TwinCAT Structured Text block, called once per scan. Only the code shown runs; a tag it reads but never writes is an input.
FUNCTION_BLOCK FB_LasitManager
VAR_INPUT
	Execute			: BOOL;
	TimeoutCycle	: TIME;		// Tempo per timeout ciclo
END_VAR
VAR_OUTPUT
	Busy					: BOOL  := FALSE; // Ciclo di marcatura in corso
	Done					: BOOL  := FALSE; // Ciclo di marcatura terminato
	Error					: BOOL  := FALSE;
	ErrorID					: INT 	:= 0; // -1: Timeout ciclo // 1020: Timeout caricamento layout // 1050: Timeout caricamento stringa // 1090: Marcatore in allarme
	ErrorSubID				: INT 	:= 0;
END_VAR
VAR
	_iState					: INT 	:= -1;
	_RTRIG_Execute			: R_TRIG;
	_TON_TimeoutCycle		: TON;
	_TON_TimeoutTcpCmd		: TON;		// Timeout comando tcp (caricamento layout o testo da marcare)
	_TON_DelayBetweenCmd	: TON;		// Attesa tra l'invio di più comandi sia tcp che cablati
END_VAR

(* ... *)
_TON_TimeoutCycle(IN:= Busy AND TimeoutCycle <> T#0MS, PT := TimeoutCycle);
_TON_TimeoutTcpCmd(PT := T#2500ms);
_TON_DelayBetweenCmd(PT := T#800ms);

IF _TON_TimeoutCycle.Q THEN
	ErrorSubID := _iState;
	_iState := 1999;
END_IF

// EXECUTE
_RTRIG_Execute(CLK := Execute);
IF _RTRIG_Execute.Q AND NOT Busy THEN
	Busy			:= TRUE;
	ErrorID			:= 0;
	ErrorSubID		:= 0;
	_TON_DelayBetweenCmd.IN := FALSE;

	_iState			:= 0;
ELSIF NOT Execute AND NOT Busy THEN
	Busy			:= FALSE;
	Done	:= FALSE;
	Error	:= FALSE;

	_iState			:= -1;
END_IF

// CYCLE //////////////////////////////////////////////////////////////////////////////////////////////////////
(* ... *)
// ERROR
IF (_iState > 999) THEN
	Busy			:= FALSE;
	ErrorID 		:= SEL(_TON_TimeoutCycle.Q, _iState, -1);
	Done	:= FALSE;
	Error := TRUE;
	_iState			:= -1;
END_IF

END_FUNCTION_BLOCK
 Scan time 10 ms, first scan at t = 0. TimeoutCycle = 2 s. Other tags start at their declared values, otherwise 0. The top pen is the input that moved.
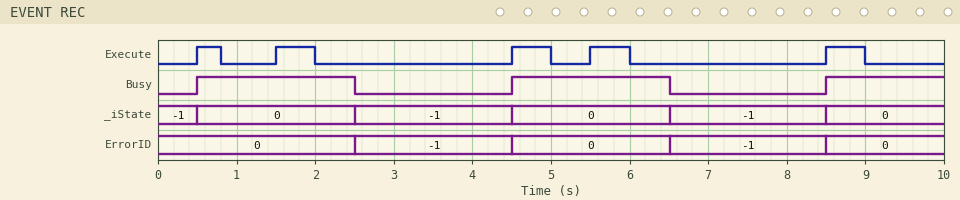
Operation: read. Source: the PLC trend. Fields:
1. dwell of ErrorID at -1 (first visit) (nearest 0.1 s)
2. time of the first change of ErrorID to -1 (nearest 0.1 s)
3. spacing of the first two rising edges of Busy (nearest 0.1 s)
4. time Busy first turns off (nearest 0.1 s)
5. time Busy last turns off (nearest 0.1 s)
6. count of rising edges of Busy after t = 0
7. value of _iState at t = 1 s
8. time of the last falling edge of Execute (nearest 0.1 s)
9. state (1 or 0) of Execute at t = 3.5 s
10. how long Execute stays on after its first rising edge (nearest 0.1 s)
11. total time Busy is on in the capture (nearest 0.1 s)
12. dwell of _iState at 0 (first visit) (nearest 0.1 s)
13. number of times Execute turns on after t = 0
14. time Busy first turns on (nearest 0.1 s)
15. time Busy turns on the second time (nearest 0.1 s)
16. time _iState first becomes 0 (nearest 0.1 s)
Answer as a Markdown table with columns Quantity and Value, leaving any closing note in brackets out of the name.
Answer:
| Quantity | Value |
|---|---|
| dwell of ErrorID at -1 (first visit) | 2.0 s |
| time of the first change of ErrorID to -1 | 2.5 s |
| spacing of the first two rising edges of Busy | 4.0 s |
| time Busy first turns off | 2.5 s |
| time Busy last turns off | 6.5 s |
| count of rising edges of Busy after t = 0 | 3 |
| value of _iState at t = 1 s | 0 |
| time of the last falling edge of Execute | 9.0 s |
| state (1 or 0) of Execute at t = 3.5 s | 0 |
| how long Execute stays on after its first rising edge | 0.3 s |
| total time Busy is on in the capture | 5.5 s |
| dwell of _iState at 0 (first visit) | 2.0 s |
| number of times Execute turns on after t = 0 | 5 |
| time Busy first turns on | 0.5 s |
| time Busy turns on the second time | 4.5 s |
| time _iState first becomes 0 | 0.5 s |
